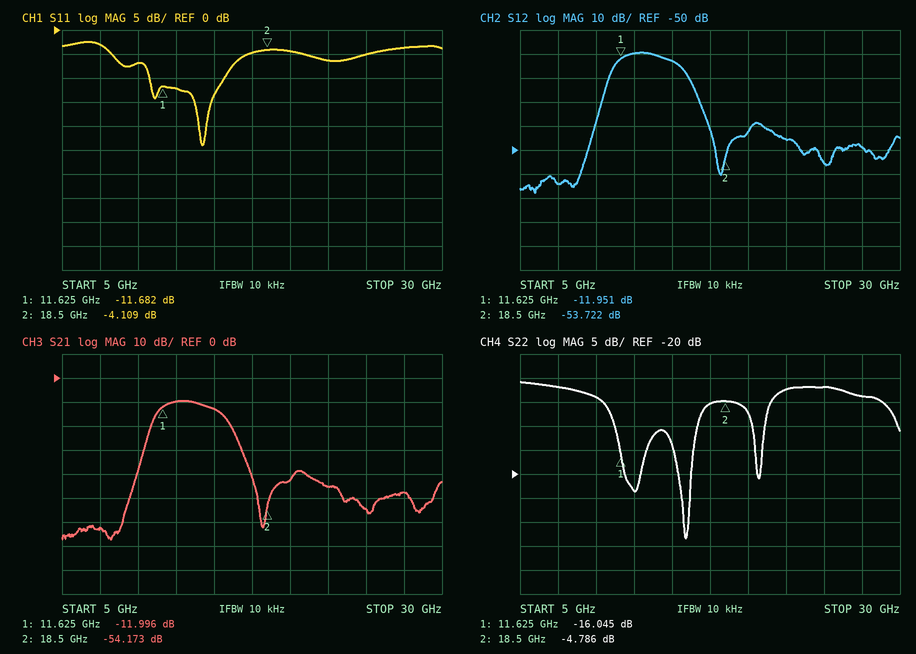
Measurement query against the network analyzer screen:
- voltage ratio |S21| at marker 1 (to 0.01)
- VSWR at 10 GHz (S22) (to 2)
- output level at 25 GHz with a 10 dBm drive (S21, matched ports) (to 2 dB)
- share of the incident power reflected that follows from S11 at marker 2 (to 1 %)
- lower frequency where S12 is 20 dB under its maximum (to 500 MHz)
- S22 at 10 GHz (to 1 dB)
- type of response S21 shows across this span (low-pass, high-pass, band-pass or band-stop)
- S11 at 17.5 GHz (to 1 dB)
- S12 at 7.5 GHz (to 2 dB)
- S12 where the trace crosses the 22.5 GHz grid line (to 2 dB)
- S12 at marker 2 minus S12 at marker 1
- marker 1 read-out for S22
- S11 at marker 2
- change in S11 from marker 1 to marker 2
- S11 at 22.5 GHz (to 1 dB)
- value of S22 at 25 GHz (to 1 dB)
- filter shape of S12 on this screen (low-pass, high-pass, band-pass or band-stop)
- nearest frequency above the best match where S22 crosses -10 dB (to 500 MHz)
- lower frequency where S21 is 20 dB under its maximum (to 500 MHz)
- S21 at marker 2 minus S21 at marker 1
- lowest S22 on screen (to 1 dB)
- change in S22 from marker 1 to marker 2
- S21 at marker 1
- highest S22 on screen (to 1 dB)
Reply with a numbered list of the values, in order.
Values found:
1. 0.25
2. 4
3. -44 dBm
4. 39 %
5. 10.5 GHz
6. -4 dB
7. band-pass
8. -5 dB
9. -64 dB
10. -46 dB
11. -41.771 dB
12. -16.045 dB
13. -4.109 dB
14. 7.573 dB
15. -6 dB
16. -2 dB
17. band-pass
18. 16.5 GHz
19. 10.5 GHz
20. -42.177 dB
21. -33 dB
22. 11.259 dB
23. -11.996 dB
24. -1 dB
